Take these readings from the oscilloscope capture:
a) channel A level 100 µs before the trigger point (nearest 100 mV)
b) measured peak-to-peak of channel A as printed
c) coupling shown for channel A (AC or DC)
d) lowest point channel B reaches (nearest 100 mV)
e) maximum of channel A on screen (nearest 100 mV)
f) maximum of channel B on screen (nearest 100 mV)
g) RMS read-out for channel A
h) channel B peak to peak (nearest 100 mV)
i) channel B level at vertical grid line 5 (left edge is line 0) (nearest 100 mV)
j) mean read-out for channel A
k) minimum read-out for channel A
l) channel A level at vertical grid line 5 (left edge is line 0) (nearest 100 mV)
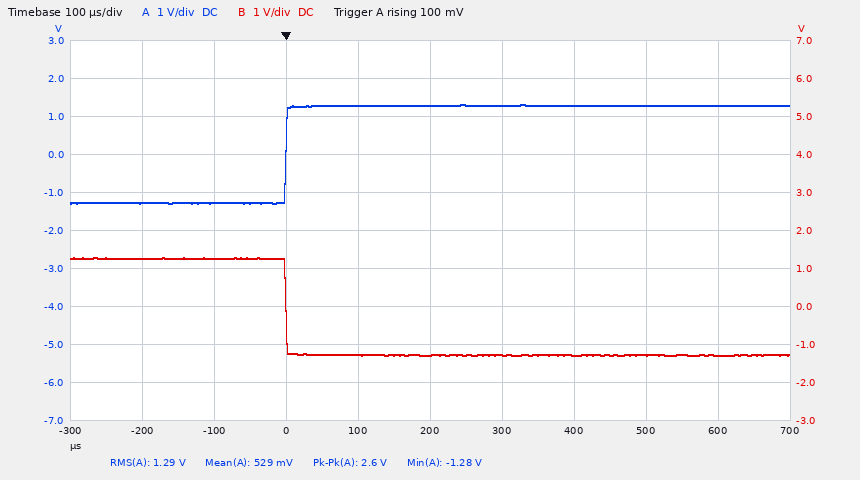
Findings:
-1.3 V
2.6 V
DC
-1.3 V
1.3 V
1.3 V
1.29 V
2.6 V
-1.3 V
529 mV
-1.28 V
1.3 V
